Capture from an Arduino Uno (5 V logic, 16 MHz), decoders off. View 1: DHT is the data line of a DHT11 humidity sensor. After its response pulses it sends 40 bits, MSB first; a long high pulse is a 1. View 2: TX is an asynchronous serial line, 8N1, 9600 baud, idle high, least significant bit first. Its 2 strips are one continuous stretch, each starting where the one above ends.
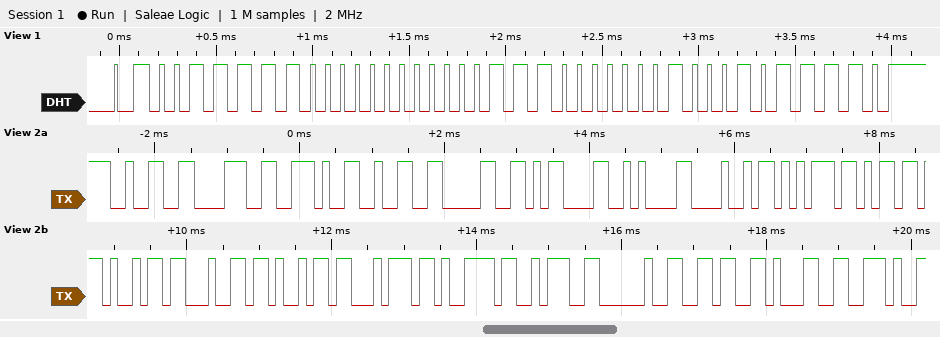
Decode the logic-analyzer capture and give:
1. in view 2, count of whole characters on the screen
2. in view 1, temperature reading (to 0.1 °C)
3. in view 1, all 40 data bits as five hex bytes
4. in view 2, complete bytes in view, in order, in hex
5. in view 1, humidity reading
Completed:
20
28.4 °C
3E 00 1C 04 5E
32 38 2E 32 30 0D 0A 48 75 6D 69 64 69 74 79 3A 20 36 31 2E
62 %
